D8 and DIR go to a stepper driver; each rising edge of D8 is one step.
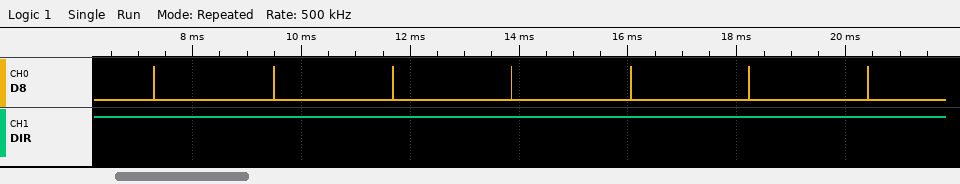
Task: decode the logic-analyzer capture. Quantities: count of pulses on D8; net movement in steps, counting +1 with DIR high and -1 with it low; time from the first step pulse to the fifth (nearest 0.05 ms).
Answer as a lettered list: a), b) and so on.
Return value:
a) 7
b) +7
c) 8.75 ms
